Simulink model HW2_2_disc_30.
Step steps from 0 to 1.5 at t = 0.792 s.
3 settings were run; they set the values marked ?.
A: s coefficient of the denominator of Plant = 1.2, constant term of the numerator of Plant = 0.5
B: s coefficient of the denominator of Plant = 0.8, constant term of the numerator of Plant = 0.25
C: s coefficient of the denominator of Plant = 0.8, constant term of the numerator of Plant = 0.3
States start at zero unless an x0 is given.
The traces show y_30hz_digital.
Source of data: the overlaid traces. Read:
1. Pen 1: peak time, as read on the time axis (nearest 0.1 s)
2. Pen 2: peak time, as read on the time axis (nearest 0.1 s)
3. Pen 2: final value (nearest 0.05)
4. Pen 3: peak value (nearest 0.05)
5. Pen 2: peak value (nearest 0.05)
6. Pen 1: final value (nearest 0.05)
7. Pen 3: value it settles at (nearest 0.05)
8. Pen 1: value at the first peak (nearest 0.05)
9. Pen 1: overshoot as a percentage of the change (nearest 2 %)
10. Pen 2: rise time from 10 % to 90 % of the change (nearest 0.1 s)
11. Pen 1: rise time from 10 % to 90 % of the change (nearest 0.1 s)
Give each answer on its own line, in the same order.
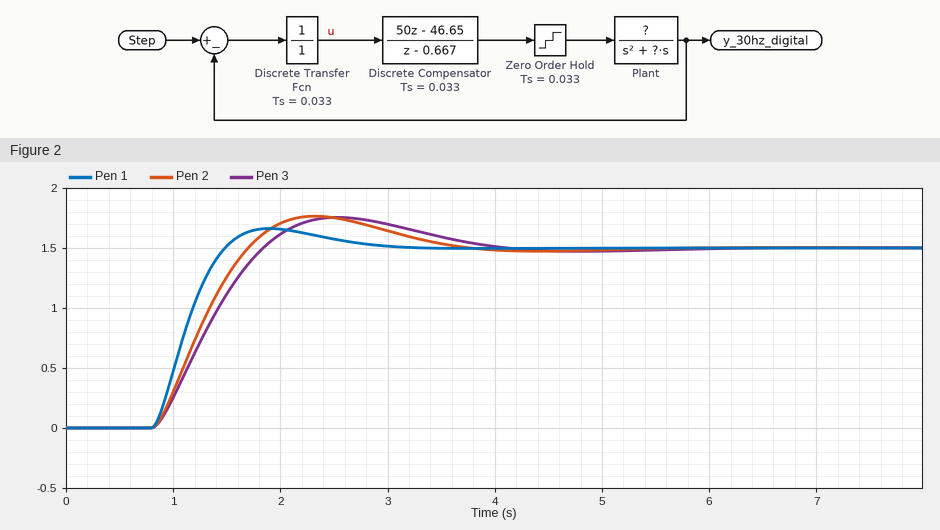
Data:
1.9 s
2.3 s
1.50
1.75
1.75
1.50
1.50
1.65
10 %
0.6 s
0.5 s
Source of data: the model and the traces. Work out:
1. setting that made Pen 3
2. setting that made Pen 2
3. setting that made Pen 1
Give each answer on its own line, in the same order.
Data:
B
C
A
